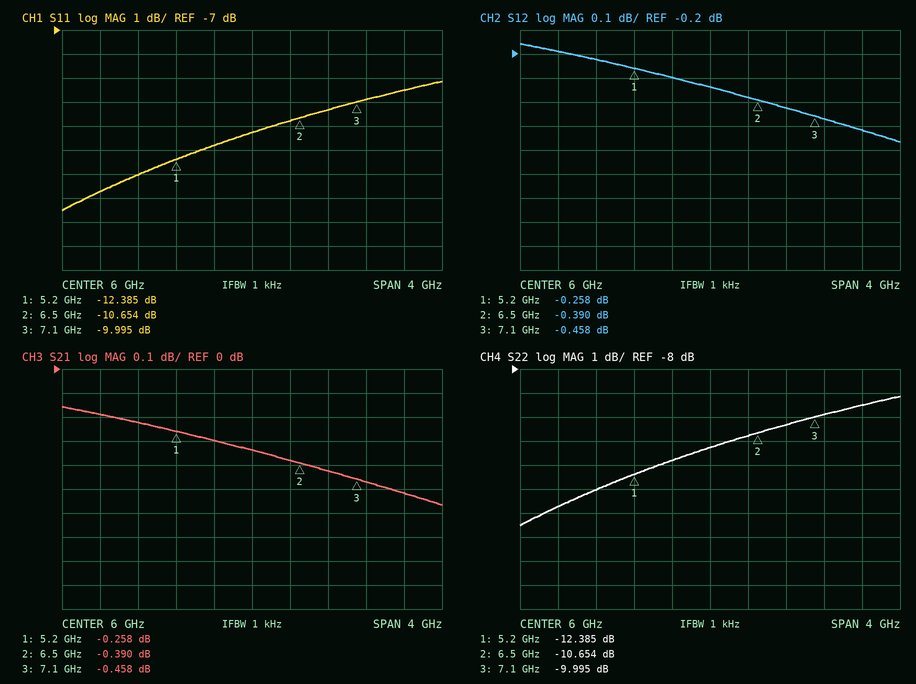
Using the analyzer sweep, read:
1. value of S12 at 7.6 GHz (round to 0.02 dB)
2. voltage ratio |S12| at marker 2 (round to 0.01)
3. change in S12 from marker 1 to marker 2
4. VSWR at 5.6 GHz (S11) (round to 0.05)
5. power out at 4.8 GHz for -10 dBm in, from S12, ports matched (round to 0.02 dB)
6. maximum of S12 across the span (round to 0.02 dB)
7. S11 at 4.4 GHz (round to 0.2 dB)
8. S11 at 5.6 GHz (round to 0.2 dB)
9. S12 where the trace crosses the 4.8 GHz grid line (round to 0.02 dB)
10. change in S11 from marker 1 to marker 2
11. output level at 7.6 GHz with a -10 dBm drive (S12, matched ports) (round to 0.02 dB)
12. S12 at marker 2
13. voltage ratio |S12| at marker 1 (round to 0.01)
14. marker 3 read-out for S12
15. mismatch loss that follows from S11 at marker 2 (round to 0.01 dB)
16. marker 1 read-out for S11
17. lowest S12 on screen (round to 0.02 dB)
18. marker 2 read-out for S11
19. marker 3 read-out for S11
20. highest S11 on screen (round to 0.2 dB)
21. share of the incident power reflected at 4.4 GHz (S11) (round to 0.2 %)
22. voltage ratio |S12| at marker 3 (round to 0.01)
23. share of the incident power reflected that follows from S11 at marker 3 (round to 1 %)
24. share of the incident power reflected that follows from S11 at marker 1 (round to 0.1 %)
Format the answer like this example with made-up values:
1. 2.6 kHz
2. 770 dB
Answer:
1. -0.52 dB
2. 0.96
3. -0.132 dB
4. 1.70
5. -10.22 dBm
6. -0.16 dB
7. -13.8 dB
8. -11.8 dB
9. -0.22 dB
10. 1.731 dB
11. -10.52 dBm
12. -0.390 dB
13. 0.97
14. -0.458 dB
15. 0.39 dB
16. -12.385 dB
17. -0.56 dB
18. -10.654 dB
19. -9.995 dB
20. -9.2 dB
21. 4.2 %
22. 0.95
23. 10 %
24. 5.8 %
